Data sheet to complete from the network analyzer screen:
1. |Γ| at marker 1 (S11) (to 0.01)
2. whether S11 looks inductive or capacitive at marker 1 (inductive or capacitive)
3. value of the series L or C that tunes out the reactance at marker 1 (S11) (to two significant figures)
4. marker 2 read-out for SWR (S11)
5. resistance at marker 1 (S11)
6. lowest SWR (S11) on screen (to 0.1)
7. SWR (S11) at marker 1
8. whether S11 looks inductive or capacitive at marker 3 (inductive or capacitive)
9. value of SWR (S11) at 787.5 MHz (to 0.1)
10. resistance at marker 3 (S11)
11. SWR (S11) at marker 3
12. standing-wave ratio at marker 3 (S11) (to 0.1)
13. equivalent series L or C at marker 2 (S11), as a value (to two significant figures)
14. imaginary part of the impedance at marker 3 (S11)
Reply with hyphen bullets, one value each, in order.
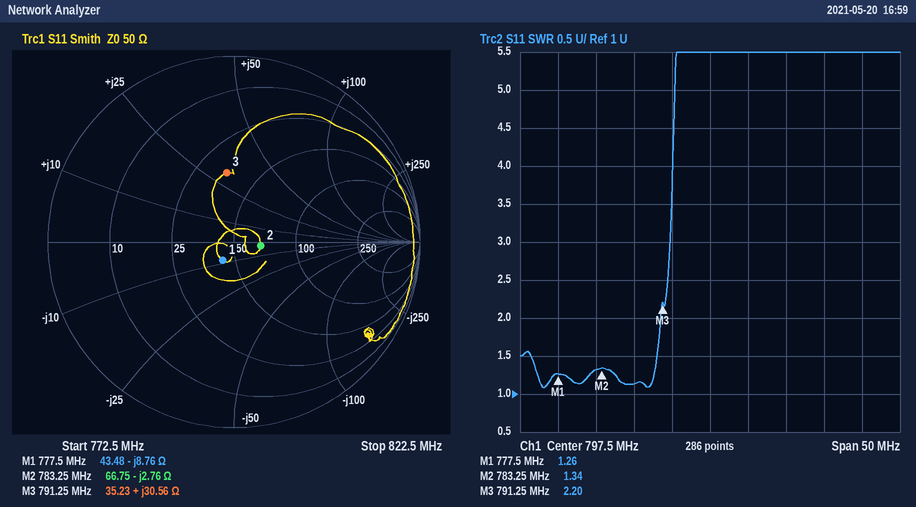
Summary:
- 0.12
- capacitive
- 1.8 nH
- 1.34
- 43.48 Ω
- 1.1
- 1.26
- inductive
- 1.1
- 35.23 Ω
- 2.20
- 2.2
- 74 pF
- +30.56 Ω
